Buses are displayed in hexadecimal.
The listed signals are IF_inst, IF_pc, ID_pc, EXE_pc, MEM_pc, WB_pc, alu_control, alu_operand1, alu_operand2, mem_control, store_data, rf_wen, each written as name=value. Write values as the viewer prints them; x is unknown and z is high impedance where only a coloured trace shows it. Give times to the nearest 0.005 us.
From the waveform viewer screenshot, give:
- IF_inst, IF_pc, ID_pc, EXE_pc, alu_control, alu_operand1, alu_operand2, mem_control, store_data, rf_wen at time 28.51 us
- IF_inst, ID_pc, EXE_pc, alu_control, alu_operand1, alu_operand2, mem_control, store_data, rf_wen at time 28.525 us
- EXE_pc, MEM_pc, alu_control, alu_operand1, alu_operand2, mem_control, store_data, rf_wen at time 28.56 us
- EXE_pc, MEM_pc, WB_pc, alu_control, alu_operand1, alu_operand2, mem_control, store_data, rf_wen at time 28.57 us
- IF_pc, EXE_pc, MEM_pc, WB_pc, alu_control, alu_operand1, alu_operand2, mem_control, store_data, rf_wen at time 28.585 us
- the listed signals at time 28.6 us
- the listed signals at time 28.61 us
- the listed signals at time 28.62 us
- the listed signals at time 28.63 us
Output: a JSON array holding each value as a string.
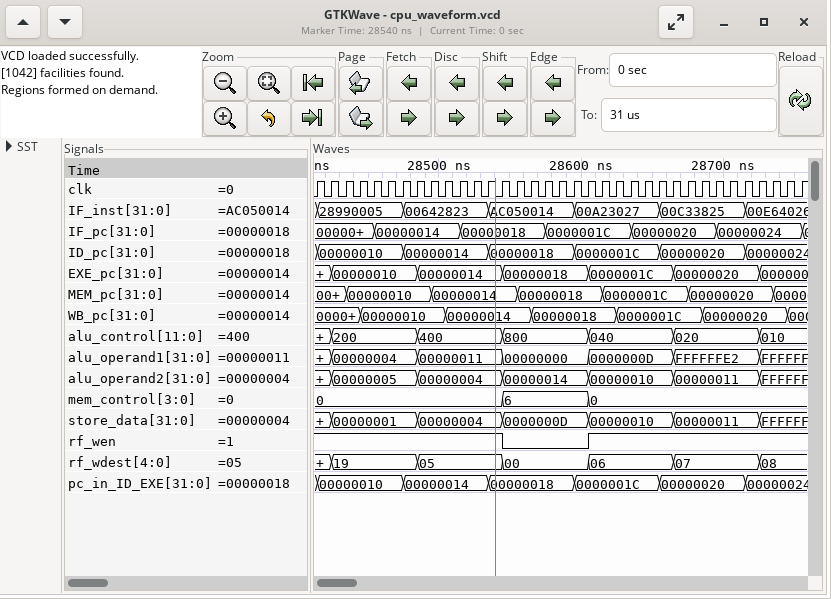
["IF_inst=00642823, IF_pc=00000014, ID_pc=00000014, EXE_pc=00000014, alu_control=400, alu_operand1=00000011, alu_operand2=00000004, mem_control=0, store_data=00000004, rf_wen=1", "IF_inst=00642823, ID_pc=00000014, EXE_pc=00000014, alu_control=400, alu_operand1=00000011, alu_operand2=00000004, mem_control=0, store_data=00000004, rf_wen=1", "EXE_pc=00000018, MEM_pc=00000018, alu_control=800, alu_operand1=00000000, alu_operand2=00000014, mem_control=6, store_data=0000000D, rf_wen=0", "EXE_pc=00000018, MEM_pc=00000018, WB_pc=00000018, alu_control=800, alu_operand1=00000000, alu_operand2=00000014, mem_control=6, store_data=0000000D, rf_wen=0", "IF_pc=0000001C, EXE_pc=00000018, MEM_pc=00000018, WB_pc=00000018, alu_control=800, alu_operand1=00000000, alu_operand2=00000014, mem_control=6, store_data=0000000D, rf_wen=0", "IF_inst=00A23027, IF_pc=0000001C, ID_pc=0000001C, EXE_pc=00000018, MEM_pc=00000018, WB_pc=00000018, alu_control=800, alu_operand1=00000000, alu_operand2=00000014, mem_control=6, store_data=0000000D, rf_wen=0", "IF_inst=00A23027, IF_pc=0000001C, ID_pc=0000001C, EXE_pc=0000001C, MEM_pc=00000018, WB_pc=00000018, alu_control=040, alu_operand1=0000000D, alu_operand2=00000010, mem_control=0, store_data=00000010, rf_wen=1", "IF_inst=00A23027, IF_pc=0000001C, ID_pc=0000001C, EXE_pc=0000001C, MEM_pc=0000001C, WB_pc=00000018, alu_control=040, alu_operand1=0000000D, alu_operand2=00000010, mem_control=0, store_data=00000010, rf_wen=1", "IF_inst=00A23027, IF_pc=0000001C, ID_pc=0000001C, EXE_pc=0000001C, MEM_pc=0000001C, WB_pc=0000001C, alu_control=040, alu_operand1=0000000D, alu_operand2=00000010, mem_control=0, store_data=00000010, rf_wen=1"]
